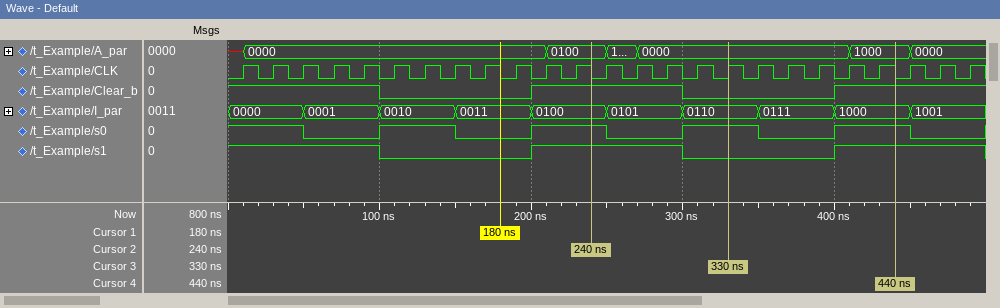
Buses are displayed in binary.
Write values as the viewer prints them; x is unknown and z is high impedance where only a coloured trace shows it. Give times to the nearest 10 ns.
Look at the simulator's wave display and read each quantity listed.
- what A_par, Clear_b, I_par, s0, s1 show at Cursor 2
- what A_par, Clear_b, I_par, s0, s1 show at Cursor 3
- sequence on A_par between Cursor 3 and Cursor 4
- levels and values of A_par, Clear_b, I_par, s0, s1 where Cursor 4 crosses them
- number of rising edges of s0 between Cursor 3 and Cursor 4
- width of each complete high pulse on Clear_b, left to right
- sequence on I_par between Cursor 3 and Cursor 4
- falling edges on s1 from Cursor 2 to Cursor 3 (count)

A_par=0100, Clear_b=1, I_par=0100, s0=1, s1=1
A_par=0000, Clear_b=0, I_par=0110, s0=1, s1=0
0000, 1000
A_par=1000, Clear_b=1, I_par=1000, s0=1, s1=1
1
100 ns
0110, 0111, 1000
1
